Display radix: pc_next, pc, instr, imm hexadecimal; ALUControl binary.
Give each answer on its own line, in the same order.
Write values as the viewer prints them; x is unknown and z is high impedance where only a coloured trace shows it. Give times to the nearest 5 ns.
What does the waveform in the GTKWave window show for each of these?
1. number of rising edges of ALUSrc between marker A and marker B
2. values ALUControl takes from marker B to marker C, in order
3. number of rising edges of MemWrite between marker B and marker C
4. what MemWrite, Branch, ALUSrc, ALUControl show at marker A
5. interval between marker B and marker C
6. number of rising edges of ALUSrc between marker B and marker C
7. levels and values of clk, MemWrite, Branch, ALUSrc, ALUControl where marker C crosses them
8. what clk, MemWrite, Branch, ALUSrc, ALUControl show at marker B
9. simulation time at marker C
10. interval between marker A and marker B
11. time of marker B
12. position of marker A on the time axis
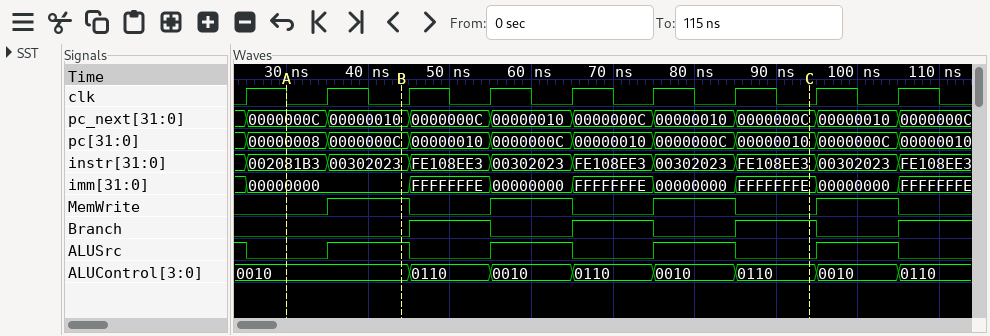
1
0010, 0110, 0010, 0110, 0010, 0110
2
MemWrite=0, Branch=0, ALUSrc=0, ALUControl=0010
50 ns
2
clk=0, MemWrite=0, Branch=1, ALUSrc=0, ALUControl=0110
clk=0, MemWrite=1, Branch=0, ALUSrc=1, ALUControl=0010
95 ns
15 ns
45 ns
30 ns
